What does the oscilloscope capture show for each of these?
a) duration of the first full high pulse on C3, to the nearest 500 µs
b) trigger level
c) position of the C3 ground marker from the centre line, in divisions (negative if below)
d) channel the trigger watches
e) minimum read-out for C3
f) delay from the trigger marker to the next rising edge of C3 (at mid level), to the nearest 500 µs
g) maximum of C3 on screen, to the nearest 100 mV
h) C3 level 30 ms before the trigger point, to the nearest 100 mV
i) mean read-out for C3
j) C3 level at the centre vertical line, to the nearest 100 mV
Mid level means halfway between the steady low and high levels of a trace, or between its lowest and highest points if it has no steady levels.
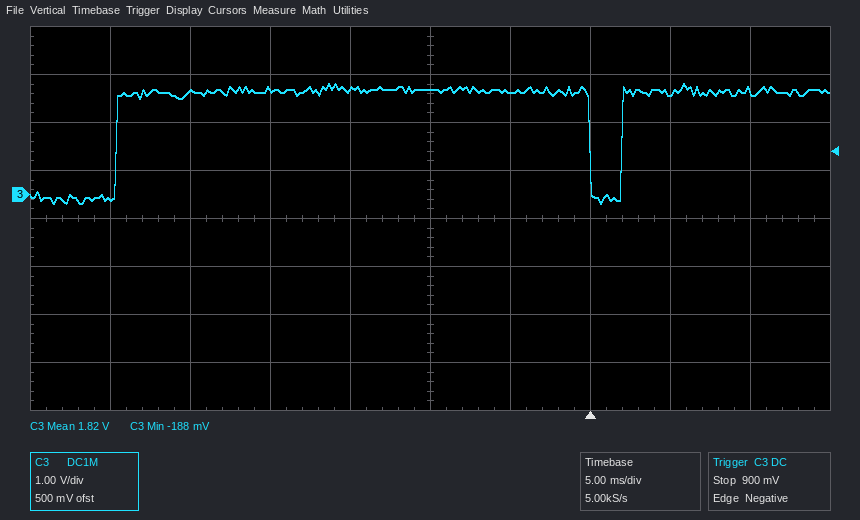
29.5 ms
900 mV
+0.5 div
C3
-188 mV
2.0 ms
2.3 V
-100 mV
1.82 V
2.2 V
